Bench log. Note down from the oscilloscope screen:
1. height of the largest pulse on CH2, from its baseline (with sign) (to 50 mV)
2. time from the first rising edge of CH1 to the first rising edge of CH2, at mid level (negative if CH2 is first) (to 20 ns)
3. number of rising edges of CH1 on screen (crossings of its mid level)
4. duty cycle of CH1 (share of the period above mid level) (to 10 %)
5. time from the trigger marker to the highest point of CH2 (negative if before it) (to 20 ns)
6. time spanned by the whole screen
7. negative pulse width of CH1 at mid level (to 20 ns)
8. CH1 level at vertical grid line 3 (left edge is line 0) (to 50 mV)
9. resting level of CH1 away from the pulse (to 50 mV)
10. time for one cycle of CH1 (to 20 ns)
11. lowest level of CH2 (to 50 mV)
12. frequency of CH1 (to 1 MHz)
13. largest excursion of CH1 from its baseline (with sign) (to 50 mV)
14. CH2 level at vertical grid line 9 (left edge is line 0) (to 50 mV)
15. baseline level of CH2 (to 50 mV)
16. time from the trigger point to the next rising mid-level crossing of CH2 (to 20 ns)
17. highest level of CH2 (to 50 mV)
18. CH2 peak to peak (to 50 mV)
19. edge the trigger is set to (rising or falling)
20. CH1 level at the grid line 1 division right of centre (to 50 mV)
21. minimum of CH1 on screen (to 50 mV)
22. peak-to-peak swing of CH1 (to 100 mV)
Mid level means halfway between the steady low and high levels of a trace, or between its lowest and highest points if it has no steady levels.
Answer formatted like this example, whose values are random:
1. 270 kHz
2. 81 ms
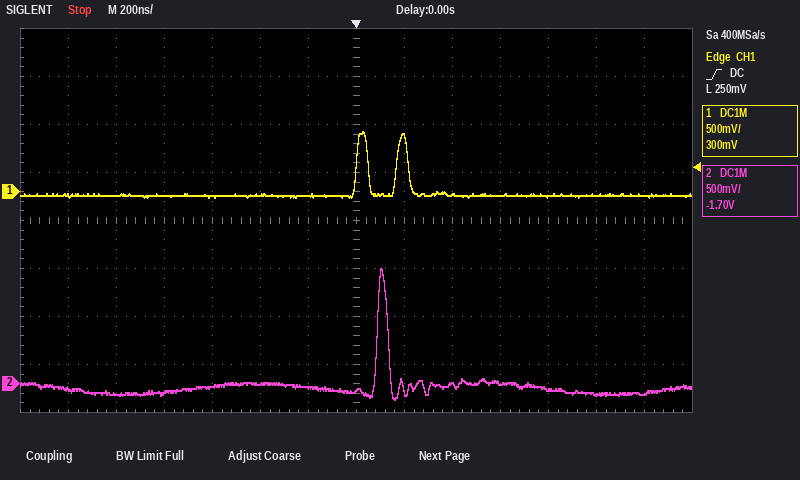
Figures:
1. +1.25 V
2. +80 ns
3. 2
4. 30 %
5. +100 ns
6. 2.8 µs
7. 120 ns
8. -50 mV
9. -50 mV
10. 160 ns
11. -150 mV
12. 6 MHz
13. +650 mV
14. 0 mV
15. -50 mV
16. 80 ns
17. 1.20 V
18. 1.35 V
19. rising
20. 550 mV
21. -50 mV
22. 700 mV
